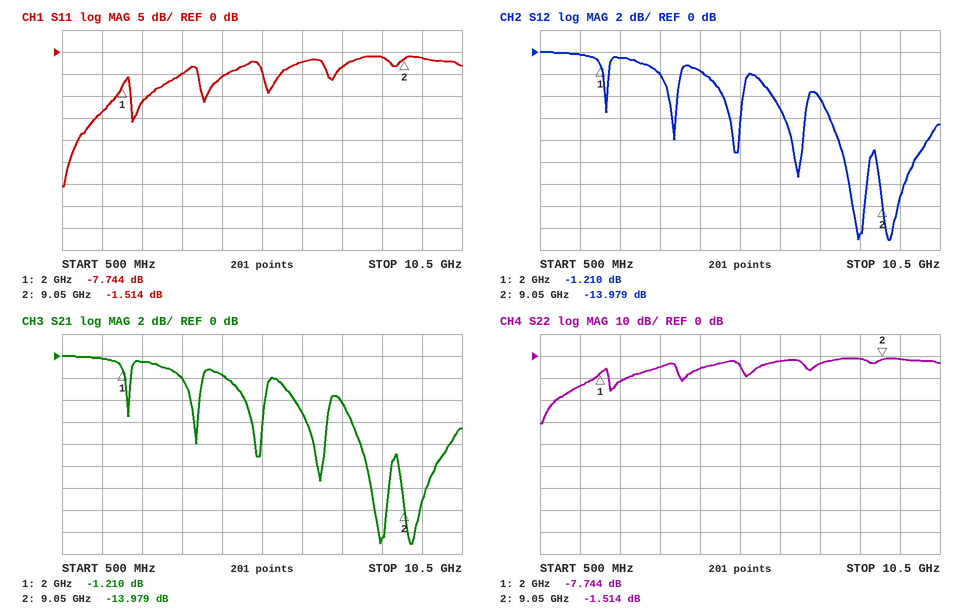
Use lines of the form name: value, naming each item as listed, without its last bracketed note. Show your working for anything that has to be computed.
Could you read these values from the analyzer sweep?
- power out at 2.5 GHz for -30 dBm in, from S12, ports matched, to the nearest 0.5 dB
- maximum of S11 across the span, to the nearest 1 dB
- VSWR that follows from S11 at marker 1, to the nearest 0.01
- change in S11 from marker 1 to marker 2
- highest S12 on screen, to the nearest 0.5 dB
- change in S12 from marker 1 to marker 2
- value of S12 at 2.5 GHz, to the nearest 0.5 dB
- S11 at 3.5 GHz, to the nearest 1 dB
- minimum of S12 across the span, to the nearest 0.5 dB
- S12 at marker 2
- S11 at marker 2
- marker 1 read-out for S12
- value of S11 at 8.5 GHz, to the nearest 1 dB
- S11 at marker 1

power out at 2.5 GHz for -30 dBm in, from S12, ports matched, to the nearest 0.5 dB: -30 dBm + (-0.5 dB) = -30.5 dBm
maximum of S11 across the span, to the nearest 1 dB: -1 dB
VSWR that follows from S11 at marker 1, to the nearest 0.01: (1 + 0.4100)/(1 − 0.4100) ≈ 2.39
change in S11 from marker 1 to marker 2: -1.514 − (-7.744) = 6.230 dB
highest S12 on screen, to the nearest 0.5 dB: 0.0 dB
change in S12 from marker 1 to marker 2: -13.979 − (-1.21) = -12.769 dB
value of S12 at 2.5 GHz, to the nearest 0.5 dB: -0.5 dB
S11 at 3.5 GHz, to the nearest 1 dB: -5 dB
minimum of S12 across the span, to the nearest 0.5 dB: -17.0 dB
S12 at marker 2: -13.979 dB
S11 at marker 2: -1.514 dB
marker 1 read-out for S12: -1.210 dB
value of S11 at 8.5 GHz, to the nearest 1 dB: -1 dB
S11 at marker 1: -7.744 dB
